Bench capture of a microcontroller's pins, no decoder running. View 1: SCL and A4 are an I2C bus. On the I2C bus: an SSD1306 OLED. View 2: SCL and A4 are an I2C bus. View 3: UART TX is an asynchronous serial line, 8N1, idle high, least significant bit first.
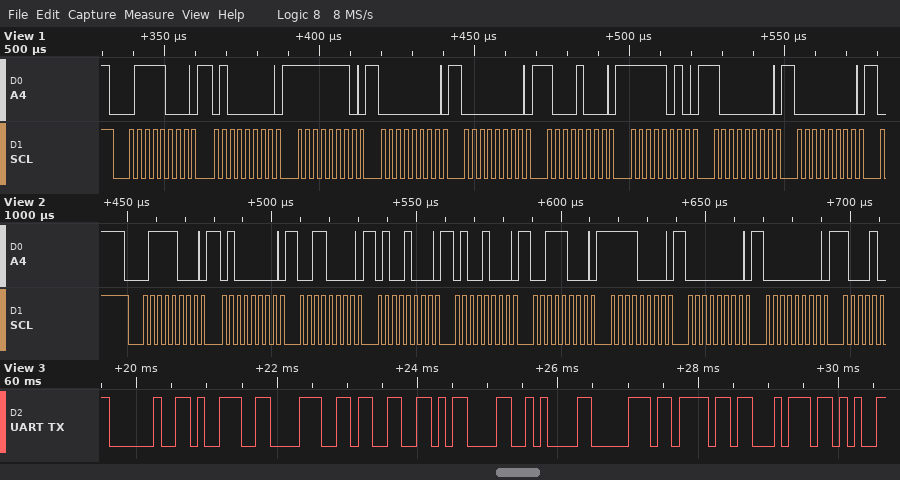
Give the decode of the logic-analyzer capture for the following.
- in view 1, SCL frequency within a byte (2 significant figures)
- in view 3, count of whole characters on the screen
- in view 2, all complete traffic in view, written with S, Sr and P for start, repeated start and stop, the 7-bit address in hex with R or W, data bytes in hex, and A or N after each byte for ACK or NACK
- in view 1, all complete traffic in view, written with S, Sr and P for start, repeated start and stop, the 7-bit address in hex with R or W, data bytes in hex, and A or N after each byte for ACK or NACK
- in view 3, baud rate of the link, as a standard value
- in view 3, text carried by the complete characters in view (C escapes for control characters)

400 kHz
9
S 3CW A 40 A 30 A 48 A 48 A 38 A F0 A 00 A 00 A
S 3CW A 40 A FE A 00 A 00 A 88 A FA A 80 A 00 A
9600 baud
" 983\r\npot"
